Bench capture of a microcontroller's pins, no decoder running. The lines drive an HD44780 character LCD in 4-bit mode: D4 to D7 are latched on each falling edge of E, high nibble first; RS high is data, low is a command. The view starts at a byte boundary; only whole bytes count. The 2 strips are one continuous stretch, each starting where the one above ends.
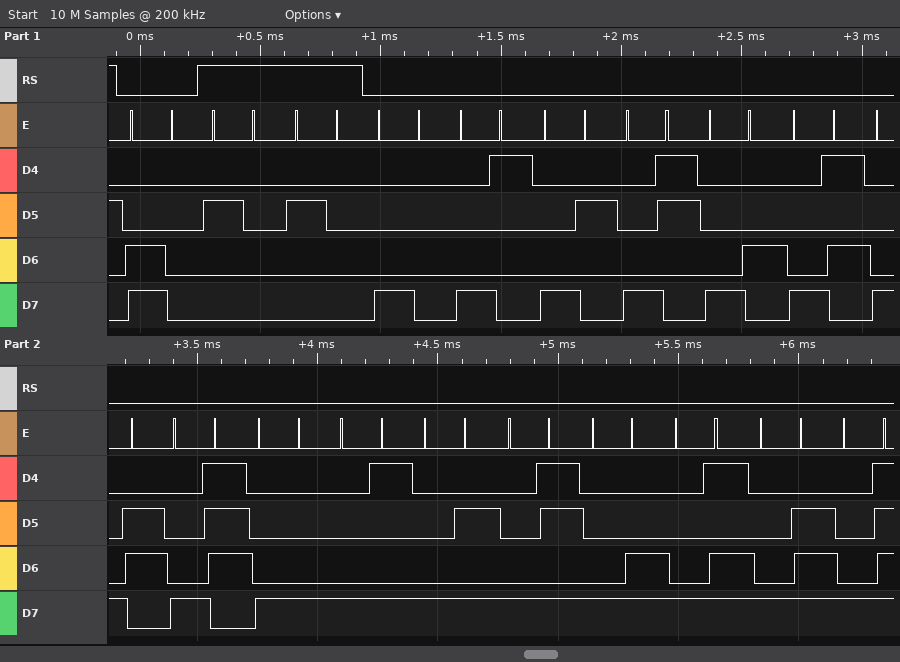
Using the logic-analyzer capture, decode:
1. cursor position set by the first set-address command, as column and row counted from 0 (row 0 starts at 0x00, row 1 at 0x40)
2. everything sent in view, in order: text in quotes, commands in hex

column 0, row 1
0xC0 "  " 0x80 0x81 0x82 0x83 0x84 0x85 0x86 0x87 0x88 0x89 0x8A 0x8B 0x8C 0x8D 0x8E 0x8F
